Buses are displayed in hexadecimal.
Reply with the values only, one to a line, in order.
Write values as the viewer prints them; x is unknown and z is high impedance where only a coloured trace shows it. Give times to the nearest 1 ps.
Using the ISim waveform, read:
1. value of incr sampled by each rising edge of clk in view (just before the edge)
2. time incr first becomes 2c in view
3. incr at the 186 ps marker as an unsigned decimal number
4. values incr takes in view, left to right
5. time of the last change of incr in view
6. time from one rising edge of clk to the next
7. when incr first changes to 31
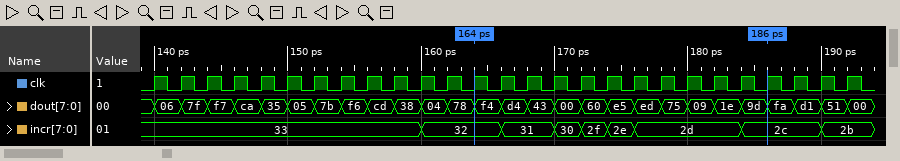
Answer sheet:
33, 33, 33, 33, 33, 33, 33, 33, 33, 33, 33, 32, 32, 32, 31, 31, 30, 2f, 2e, 2d, 2d, 2d, 2d, 2c, 2c, 2c, 2b
184 ps
44
33, 32, 31, 30, 2f, 2e, 2d, 2c, 2b
190 ps
2 ps
166 ps
